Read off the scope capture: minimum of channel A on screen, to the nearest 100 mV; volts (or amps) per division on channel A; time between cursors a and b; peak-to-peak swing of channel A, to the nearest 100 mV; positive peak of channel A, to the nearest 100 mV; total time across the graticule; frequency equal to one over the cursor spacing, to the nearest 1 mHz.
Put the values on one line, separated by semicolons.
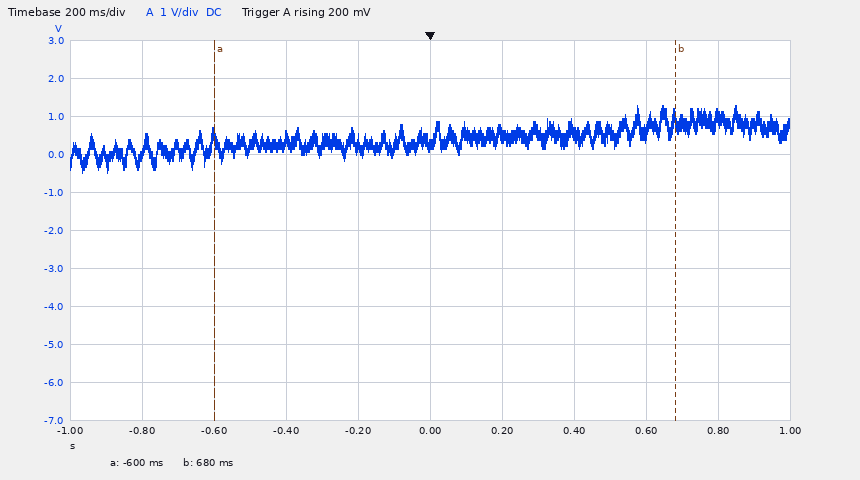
-500 mV; 1 V; 1.28 s; 1.8 V; 1.3 V; 2 s; 781 mHz
